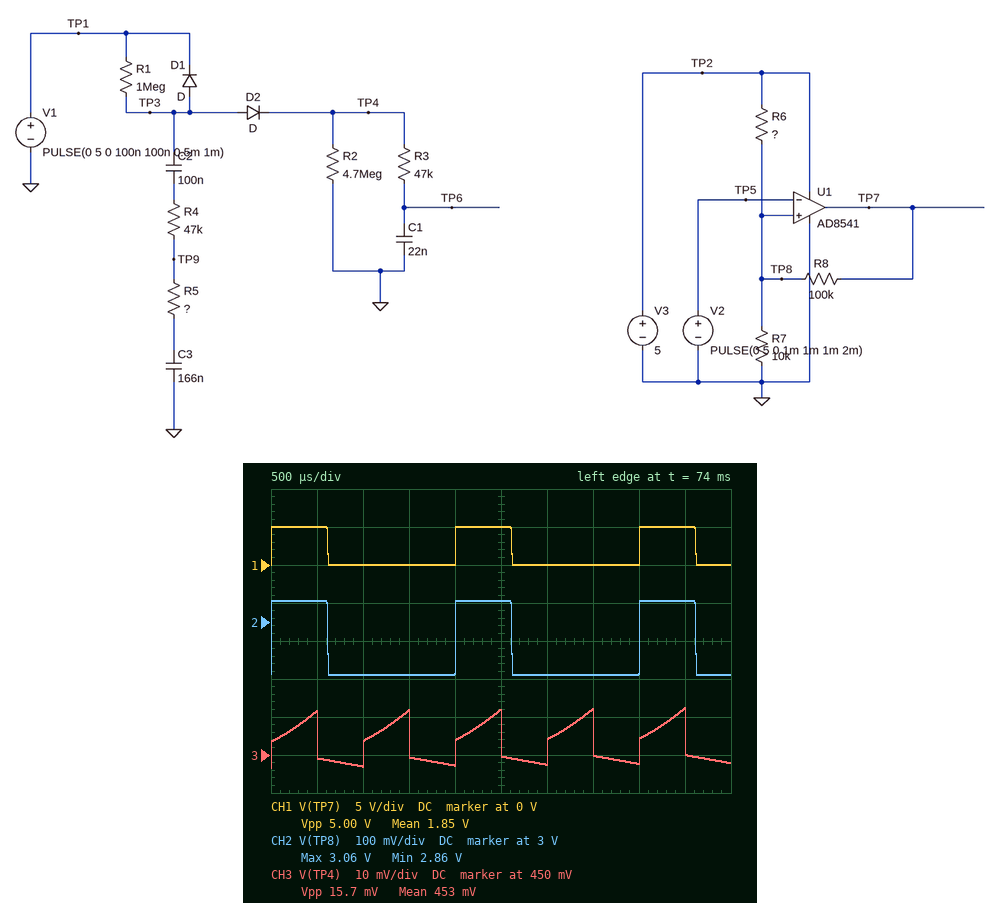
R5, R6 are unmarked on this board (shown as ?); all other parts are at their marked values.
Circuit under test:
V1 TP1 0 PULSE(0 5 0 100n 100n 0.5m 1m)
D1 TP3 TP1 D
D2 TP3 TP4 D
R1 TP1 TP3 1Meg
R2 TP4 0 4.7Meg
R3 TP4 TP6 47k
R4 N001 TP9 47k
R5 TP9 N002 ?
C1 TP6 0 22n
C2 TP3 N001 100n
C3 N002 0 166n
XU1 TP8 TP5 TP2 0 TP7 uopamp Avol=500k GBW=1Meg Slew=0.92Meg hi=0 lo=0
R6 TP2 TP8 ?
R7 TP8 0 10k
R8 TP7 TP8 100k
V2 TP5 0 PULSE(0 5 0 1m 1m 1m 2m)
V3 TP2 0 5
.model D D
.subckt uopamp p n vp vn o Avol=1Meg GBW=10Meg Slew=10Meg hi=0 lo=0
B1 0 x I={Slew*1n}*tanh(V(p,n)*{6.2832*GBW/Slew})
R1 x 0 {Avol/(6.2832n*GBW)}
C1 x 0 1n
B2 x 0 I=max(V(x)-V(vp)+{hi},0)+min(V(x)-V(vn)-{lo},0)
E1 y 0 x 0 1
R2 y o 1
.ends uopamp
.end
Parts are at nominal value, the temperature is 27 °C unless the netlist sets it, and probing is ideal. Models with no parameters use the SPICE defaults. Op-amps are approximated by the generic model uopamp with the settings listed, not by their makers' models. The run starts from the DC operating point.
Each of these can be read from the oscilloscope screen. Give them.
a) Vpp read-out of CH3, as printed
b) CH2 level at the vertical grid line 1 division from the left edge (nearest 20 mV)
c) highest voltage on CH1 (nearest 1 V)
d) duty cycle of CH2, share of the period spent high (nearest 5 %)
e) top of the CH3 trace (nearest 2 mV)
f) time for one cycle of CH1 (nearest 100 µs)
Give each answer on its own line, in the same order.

15.7 mV
3.06 V
5 V
30 %
462 mV
2.0 ms
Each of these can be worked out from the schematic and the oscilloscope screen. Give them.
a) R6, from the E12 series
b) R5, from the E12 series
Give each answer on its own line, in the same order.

6.8 kΩ
2.2 kΩ
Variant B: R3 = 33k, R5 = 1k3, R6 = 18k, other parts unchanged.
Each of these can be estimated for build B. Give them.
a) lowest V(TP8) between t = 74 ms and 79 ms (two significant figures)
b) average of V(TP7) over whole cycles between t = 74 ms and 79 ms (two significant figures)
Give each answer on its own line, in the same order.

1.7 V
1.0 V
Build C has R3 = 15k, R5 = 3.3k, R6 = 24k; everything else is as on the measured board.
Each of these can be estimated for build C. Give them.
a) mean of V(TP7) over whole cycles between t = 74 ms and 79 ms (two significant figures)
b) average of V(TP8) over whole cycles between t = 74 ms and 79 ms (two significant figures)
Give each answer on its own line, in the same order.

860 mV
1.4 V
